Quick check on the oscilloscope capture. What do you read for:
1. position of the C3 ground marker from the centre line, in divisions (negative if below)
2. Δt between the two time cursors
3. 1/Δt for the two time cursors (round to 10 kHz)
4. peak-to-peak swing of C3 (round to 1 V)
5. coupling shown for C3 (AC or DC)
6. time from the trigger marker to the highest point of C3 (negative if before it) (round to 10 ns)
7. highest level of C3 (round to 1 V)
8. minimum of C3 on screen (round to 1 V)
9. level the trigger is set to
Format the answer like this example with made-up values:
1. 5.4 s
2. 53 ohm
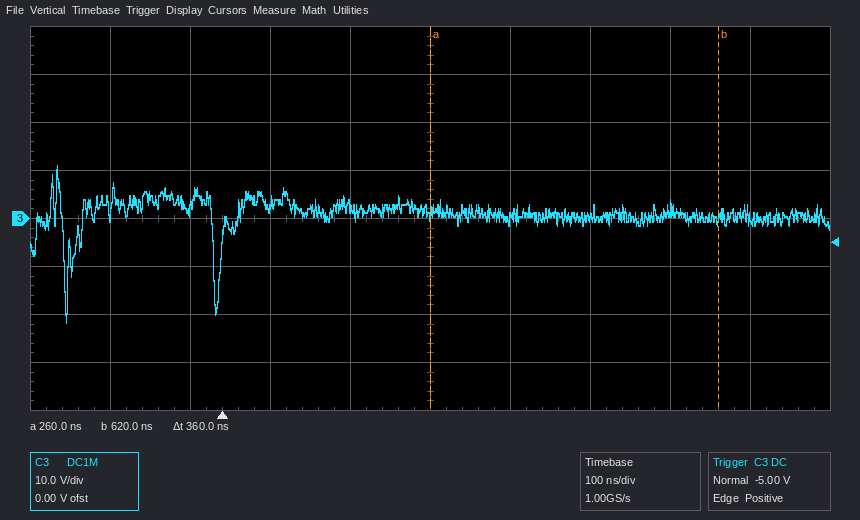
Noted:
1. 0.0 div
2. 360 ns
3. 2.78 MHz
4. 33 V
5. DC
6. -210 ns
7. 11 V
8. -22 V
9. -5.00 V
